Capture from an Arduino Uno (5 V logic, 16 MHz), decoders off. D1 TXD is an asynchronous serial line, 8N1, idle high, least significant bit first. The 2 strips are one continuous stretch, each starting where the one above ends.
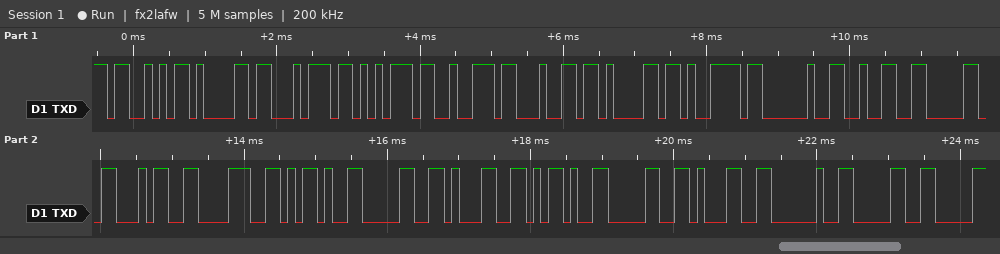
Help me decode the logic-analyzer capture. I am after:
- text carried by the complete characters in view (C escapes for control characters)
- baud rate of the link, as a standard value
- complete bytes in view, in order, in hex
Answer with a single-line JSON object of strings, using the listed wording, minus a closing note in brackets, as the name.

{"text carried by the complete characters in view": "\"Saturday 2048-01-01 0\"", "baud rate of the link, as a standard value": "9600 baud", "complete bytes in view, in order, in hex": "53 61 74 75 72 64 61 79 20 32 30 34 38 2D 30 31 2D 30 31 20 30"}
